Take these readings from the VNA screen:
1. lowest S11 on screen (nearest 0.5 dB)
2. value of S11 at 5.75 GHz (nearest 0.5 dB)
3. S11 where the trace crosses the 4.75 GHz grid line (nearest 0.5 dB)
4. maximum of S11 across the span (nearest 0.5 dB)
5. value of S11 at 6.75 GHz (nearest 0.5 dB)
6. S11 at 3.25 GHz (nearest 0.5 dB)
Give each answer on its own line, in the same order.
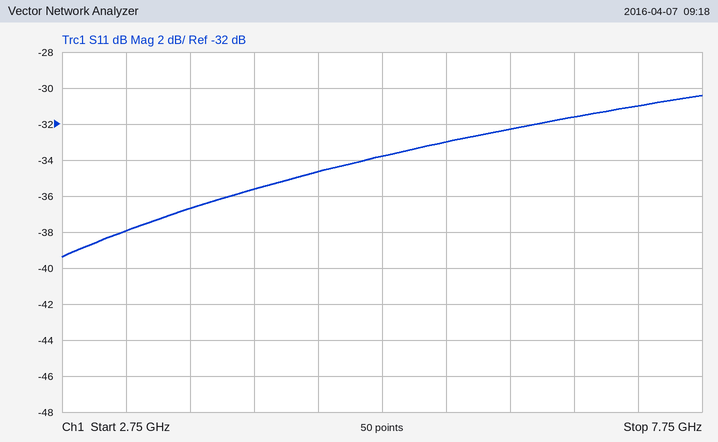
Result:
-39.5 dB
-33.0 dB
-34.5 dB
-30.5 dB
-31.5 dB
-38.0 dB
